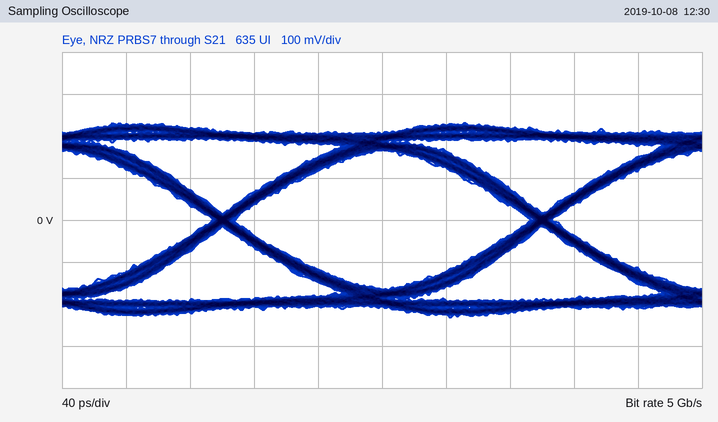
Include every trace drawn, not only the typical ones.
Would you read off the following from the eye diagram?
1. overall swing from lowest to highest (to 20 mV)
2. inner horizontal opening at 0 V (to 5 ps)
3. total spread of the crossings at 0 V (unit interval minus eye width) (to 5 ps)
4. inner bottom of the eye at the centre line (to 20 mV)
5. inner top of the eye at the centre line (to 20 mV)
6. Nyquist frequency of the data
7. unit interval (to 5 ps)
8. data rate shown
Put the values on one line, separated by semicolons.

460 mV; 185 ps; 15 ps; -160 mV; 160 mV; 2.5 GHz; 200 ps; 5 Gb/s
